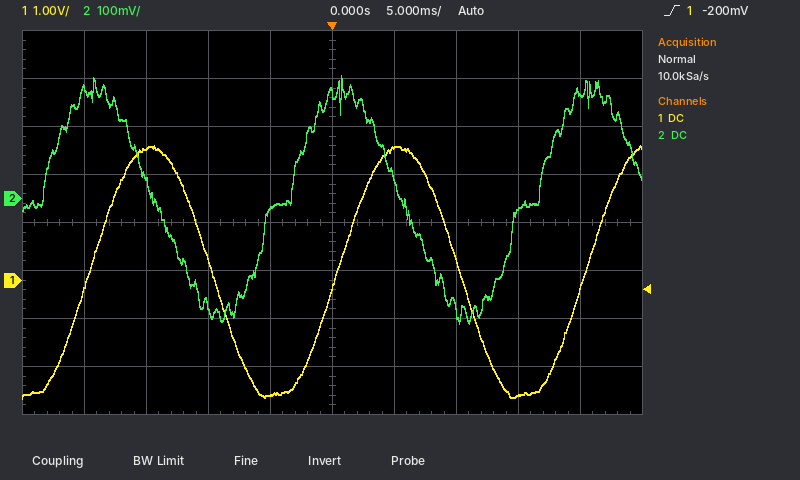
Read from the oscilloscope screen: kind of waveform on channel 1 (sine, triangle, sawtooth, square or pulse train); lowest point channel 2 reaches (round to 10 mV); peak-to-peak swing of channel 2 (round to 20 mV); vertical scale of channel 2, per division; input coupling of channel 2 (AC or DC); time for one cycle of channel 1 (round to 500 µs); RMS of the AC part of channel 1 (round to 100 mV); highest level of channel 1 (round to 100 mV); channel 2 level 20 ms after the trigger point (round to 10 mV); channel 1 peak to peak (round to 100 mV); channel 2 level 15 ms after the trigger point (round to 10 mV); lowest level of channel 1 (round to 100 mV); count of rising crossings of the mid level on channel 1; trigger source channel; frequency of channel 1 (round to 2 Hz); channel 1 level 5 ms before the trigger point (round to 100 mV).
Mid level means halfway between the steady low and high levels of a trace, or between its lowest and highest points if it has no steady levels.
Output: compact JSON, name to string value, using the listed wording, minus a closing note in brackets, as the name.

{"kind of waveform on channel 1": "sine", "lowest point channel 2 reaches": "-260 mV", "peak-to-peak swing of channel 2": "520 mV", "vertical scale of channel 2, per division": "100 mV", "input coupling of channel 2": "DC", "time for one cycle of channel 1": "20.0 ms", "RMS of the AC part of channel 1": "1.9 V", "highest level of channel 1": "2.8 V", "channel 2 level 20 ms after the trigger point": "220 mV", "channel 1 peak to peak": "5.3 V", "channel 2 level 15 ms after the trigger point": "-30 mV", "lowest level of channel 1": "-2.5 V", "count of rising crossings of the mid level on channel 1": "3", "trigger source channel": "channel 1", "frequency of channel 1": "50 Hz", "channel 1 level 5 ms before the trigger point": "-2.4 V"}
